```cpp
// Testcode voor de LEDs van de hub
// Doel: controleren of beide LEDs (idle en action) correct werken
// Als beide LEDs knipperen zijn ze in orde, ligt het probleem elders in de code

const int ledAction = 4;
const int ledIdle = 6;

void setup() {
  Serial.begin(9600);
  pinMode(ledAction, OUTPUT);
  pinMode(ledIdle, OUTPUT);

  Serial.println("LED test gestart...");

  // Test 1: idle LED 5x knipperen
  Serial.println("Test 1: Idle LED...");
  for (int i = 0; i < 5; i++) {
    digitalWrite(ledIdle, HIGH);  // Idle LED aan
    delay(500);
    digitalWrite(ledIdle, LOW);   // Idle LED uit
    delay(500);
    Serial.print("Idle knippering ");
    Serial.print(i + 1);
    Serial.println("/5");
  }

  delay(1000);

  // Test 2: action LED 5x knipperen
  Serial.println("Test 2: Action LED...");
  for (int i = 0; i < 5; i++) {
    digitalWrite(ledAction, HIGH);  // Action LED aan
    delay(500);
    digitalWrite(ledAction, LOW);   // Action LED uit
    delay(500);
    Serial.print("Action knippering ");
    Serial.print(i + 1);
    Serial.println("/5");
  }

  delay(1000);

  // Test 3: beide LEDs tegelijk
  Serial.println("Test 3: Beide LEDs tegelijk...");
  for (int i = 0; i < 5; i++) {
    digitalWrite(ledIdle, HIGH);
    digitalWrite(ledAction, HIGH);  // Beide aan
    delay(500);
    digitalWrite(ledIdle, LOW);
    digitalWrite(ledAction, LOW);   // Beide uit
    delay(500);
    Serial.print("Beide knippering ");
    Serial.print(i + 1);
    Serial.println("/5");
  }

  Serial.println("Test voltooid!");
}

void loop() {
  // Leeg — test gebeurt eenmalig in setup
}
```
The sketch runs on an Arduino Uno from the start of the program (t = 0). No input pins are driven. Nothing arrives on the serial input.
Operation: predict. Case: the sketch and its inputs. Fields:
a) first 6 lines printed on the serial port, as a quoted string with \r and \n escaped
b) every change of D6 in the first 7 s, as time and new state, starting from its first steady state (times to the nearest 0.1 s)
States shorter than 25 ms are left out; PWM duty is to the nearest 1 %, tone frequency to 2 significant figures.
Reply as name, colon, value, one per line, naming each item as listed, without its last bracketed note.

first 6 lines printed on the serial port, as a quoted string with \r and \n escaped: "LED test gestart...\r\nTest 1: Idle LED...\r\nIdle knippering 1/5\r\nIdle knippering 2/5\r\nIdle knippering 3/5\r\nIdle knippering 4/5\r\n"
every change of D6 in the first 7 s, as time and new state, starting from its first steady state: 0 s high; 0.5 s low; 1 s high; 1.5 s low; 2 s high; 2.5 s low; 3 s high; 3.5 s low; 4 s high; 4.5 s low
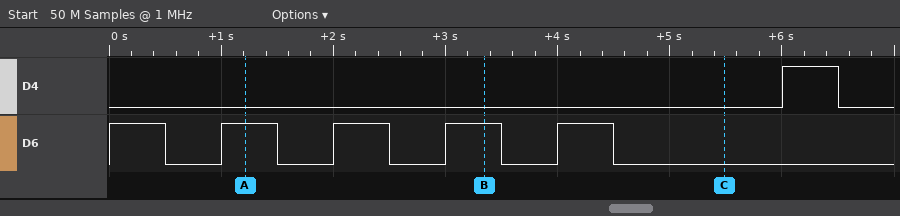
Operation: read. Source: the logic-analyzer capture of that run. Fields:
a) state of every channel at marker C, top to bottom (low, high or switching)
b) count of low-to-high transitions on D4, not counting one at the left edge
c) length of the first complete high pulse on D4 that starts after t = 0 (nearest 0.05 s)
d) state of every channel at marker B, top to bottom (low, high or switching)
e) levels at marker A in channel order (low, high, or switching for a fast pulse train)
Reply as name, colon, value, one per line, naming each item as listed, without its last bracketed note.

state of every channel at marker C, top to bottom: D4 low, D6 low
count of low-to-high transitions on D4, not counting one at the left edge: 1
length of the first complete high pulse on D4 that starts after t = 0: 0.50 s
state of every channel at marker B, top to bottom: D4 low, D6 high
levels at marker A in channel order: D4 low, D6 high
